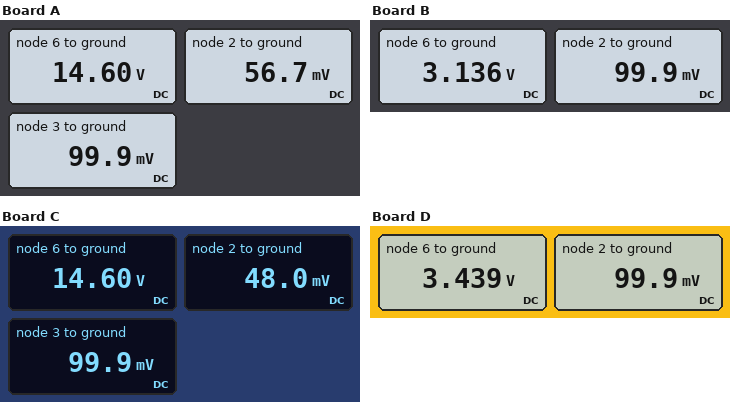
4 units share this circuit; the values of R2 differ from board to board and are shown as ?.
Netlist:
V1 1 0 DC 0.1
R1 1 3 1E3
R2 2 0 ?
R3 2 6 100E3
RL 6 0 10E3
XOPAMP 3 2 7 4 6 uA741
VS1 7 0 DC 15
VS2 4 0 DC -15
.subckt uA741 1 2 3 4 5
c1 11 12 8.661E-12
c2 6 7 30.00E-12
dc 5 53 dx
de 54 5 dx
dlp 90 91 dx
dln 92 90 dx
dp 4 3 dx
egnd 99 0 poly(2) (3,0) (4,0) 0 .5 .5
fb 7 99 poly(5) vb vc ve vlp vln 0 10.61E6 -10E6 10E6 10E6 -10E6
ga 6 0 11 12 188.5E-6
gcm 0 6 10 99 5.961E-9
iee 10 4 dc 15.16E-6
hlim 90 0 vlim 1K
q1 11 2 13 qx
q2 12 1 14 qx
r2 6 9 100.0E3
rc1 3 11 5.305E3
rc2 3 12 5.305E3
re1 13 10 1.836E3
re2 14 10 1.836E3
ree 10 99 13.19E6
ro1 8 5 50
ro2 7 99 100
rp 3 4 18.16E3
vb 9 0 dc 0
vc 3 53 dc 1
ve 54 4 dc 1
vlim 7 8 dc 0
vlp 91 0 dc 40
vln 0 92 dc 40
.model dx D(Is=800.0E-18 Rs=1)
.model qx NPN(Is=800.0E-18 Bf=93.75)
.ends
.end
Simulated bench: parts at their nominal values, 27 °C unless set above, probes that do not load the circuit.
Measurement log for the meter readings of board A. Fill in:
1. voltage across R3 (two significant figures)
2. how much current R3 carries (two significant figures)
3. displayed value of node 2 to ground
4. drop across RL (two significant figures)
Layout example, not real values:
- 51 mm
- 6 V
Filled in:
- 15 V
- 150 µA
- 56.7 mV
- 15 V
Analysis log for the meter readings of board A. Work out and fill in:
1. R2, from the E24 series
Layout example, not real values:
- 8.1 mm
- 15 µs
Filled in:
- 390 Ω
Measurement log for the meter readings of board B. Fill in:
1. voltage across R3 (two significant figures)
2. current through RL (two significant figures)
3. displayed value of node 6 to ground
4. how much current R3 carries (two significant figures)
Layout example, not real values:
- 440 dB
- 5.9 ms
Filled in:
- 3.0 V
- 310 µA
- 3.136 V
- 30 µA
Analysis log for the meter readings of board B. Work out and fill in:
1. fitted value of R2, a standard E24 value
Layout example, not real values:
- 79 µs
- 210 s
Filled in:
- 3.3 kΩ
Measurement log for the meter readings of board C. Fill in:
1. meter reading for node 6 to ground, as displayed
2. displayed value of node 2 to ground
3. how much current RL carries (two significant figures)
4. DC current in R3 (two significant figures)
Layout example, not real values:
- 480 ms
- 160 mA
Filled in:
- 14.60 V
- 48.0 mV
- 1.5 mA
- 150 µA
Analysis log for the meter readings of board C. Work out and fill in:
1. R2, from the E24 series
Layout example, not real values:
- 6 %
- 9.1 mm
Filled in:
- 330 Ω
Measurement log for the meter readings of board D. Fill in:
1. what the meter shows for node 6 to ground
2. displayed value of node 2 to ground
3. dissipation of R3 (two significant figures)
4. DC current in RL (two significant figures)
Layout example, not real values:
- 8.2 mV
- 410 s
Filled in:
- 3.439 V
- 99.9 mV
- 110 µW
- 340 µA
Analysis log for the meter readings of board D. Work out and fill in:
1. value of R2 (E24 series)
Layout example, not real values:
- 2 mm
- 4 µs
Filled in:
- 3 kΩ
